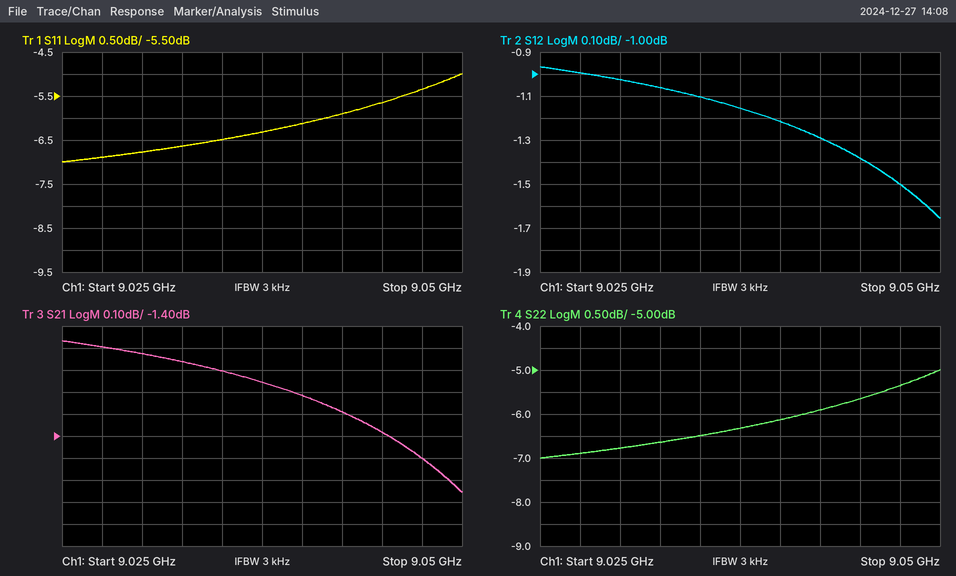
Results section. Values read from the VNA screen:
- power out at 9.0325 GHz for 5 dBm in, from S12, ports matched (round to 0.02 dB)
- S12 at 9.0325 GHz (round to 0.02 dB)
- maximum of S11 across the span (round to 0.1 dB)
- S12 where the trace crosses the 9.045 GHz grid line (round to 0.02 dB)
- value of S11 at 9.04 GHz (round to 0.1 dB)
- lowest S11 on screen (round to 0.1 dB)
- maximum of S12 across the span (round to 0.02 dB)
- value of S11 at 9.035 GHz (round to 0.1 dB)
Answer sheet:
3.94 dBm
-1.06 dB
-5.0 dB
-1.38 dB
-6.1 dB
-7.0 dB
-0.96 dB
-6.5 dB
